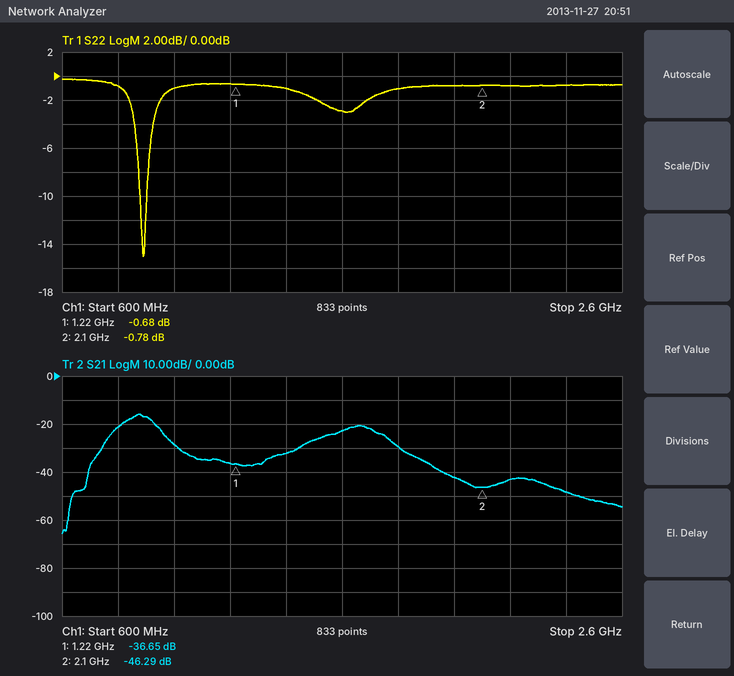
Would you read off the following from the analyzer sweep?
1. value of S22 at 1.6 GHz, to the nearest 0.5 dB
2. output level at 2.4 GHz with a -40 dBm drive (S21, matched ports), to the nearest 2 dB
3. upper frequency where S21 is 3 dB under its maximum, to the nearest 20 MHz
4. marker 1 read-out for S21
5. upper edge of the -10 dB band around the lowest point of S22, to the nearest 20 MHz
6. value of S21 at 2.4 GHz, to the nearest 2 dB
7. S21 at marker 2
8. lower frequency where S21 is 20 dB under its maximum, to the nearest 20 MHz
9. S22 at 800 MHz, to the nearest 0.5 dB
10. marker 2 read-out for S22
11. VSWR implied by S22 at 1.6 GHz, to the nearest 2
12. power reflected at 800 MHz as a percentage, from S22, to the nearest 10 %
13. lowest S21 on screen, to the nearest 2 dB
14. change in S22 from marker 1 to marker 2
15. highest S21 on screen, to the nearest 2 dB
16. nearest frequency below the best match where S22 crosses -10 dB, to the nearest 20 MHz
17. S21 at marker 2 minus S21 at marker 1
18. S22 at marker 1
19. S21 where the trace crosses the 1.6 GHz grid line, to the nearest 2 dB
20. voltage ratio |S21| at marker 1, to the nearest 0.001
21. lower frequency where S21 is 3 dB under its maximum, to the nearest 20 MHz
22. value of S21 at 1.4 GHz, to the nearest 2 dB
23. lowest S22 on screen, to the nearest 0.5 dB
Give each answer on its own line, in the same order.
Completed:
-3.0 dB
-88 dBm
920 MHz
-36.65 dB
900 MHz
-48 dB
-46.29 dB
700 MHz
-1.0 dB
-0.78 dB
6
80 %
-66 dB
-0.10 dB
-16 dB
880 MHz
-9.64 dB
-0.68 dB
-22 dB
0.015
820 MHz
-32 dB
-15.0 dB
